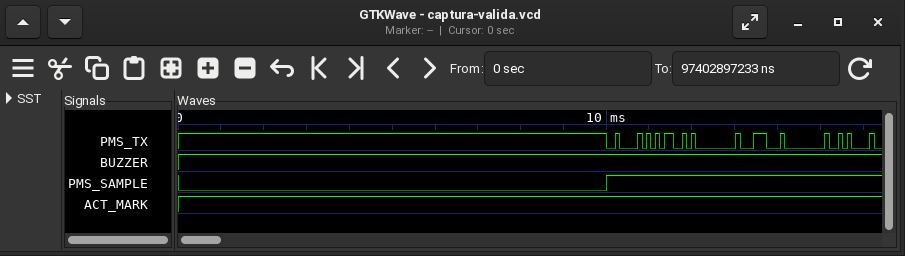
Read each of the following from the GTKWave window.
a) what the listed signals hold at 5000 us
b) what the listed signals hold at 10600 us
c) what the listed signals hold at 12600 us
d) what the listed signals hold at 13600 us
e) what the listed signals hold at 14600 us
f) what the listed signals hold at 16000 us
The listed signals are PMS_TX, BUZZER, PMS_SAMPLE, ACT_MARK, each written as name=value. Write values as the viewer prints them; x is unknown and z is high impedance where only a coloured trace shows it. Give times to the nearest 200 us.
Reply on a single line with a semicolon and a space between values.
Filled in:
PMS_TX=1, BUZZER=1, PMS_SAMPLE=0, ACT_MARK=1; PMS_TX=0, BUZZER=1, PMS_SAMPLE=1, ACT_MARK=1; PMS_TX=0, BUZZER=1, PMS_SAMPLE=1, ACT_MARK=1; PMS_TX=1, BUZZER=1, PMS_SAMPLE=1, ACT_MARK=1; PMS_TX=0, BUZZER=1, PMS_SAMPLE=1, ACT_MARK=1; PMS_TX=0, BUZZER=1, PMS_SAMPLE=1, ACT_MARK=1
